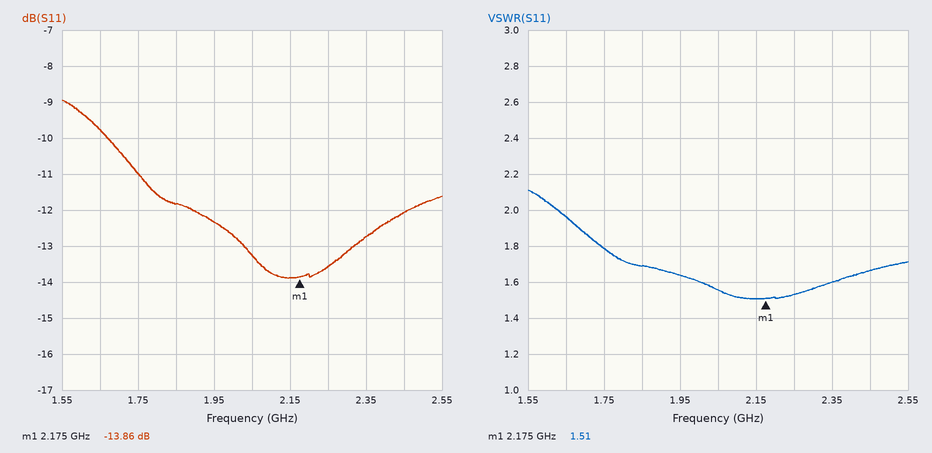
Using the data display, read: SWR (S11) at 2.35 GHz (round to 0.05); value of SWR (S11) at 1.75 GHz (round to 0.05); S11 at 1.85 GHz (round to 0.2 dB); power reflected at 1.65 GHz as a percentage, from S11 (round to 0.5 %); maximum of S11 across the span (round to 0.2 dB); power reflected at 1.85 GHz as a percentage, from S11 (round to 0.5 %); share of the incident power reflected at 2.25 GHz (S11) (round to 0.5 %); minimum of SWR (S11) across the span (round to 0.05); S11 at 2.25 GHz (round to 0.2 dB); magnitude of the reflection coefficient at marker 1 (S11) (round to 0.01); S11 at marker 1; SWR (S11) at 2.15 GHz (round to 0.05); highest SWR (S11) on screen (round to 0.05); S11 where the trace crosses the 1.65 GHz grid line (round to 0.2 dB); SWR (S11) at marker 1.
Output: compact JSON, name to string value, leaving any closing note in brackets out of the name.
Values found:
{"SWR (S11) at 2.35 GHz": "1.60", "value of SWR (S11) at 1.75 GHz": "1.80", "S11 at 1.85 GHz": "-11.8 dB", "power reflected at 1.65 GHz as a percentage, from S11": "10.5 %", "maximum of S11 across the span": "-9.0 dB", "power reflected at 1.85 GHz as a percentage, from S11": "6.5 %", "share of the incident power reflected at 2.25 GHz (S11)": "4.5 %", "minimum of SWR (S11) across the span": "1.50", "S11 at 2.25 GHz": "-13.6 dB", "magnitude of the reflection coefficient at marker 1 (S11)": "0.20", "S11 at marker 1": "-13.86 dB", "SWR (S11) at 2.15 GHz": "1.50", "highest SWR (S11) on screen": "2.10", "S11 where the trace crosses the 1.65 GHz grid line": "-9.8 dB", "SWR (S11) at marker 1": "1.51"}
